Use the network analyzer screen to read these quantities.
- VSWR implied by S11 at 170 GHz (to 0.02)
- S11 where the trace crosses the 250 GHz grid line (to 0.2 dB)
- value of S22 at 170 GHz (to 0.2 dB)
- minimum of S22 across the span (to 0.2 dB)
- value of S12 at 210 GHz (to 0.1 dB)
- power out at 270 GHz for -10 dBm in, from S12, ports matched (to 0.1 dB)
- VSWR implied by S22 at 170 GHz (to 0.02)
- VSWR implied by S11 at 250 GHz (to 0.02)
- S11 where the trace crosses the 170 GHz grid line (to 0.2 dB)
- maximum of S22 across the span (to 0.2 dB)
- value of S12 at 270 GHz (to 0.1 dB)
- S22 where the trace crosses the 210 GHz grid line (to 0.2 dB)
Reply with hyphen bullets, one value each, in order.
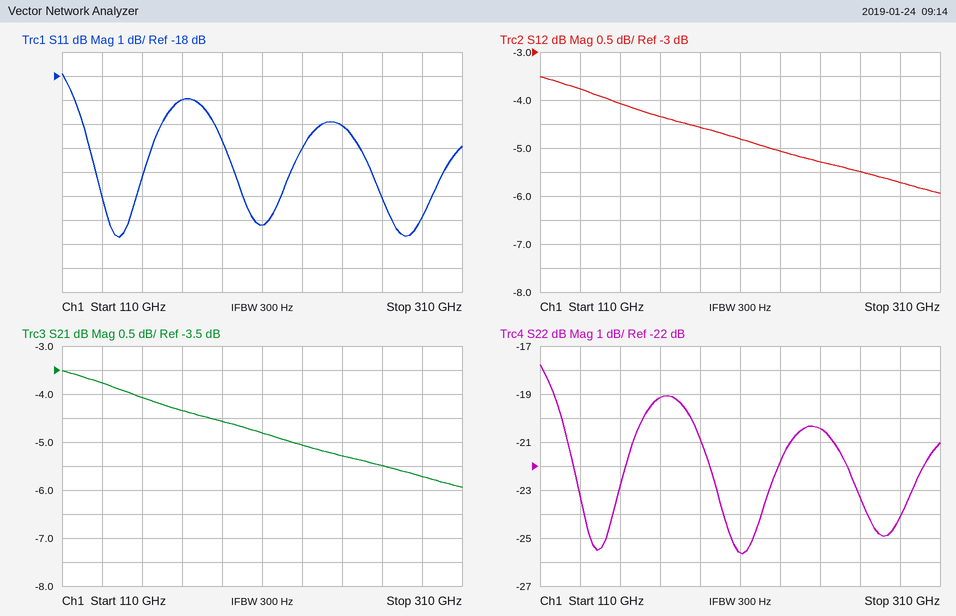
- 1.26
- -20.0 dB
- -19.2 dB
- -25.6 dB
- -4.8 dB
- -15.5 dBm
- 1.24
- 1.22
- -19.0 dB
- -17.8 dB
- -5.5 dB
- -25.6 dB
